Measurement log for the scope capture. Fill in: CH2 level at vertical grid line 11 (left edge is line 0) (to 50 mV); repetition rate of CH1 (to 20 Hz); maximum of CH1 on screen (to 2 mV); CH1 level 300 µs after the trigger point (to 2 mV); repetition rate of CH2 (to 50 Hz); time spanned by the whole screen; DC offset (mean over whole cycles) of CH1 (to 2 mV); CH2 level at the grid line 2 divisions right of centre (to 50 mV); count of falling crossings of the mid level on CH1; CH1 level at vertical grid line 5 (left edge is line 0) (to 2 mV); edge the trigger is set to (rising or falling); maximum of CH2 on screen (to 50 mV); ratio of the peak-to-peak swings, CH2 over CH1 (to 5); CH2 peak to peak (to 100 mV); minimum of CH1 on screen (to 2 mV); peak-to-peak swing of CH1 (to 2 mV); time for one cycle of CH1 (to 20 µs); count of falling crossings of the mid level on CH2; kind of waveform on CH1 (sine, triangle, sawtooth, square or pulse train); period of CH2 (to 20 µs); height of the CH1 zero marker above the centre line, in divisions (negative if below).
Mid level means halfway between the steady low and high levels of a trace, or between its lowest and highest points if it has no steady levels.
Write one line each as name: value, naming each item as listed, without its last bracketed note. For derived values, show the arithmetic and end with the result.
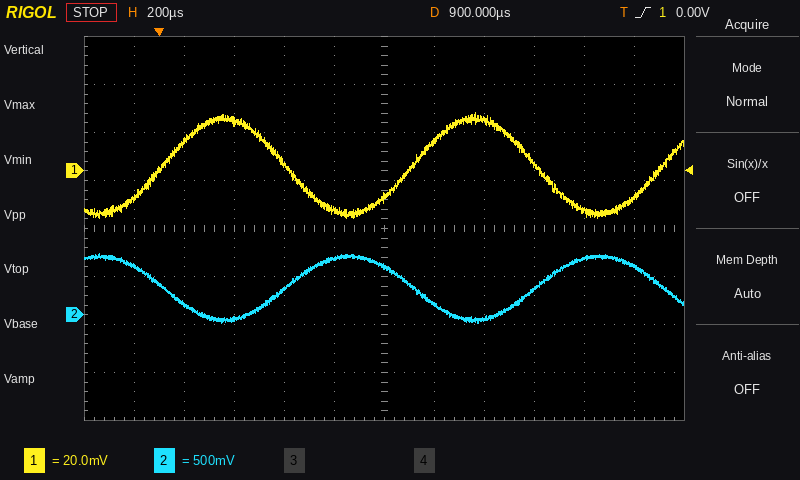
CH2 level at vertical grid line 11 (left edge is line 0): 500 mV
repetition rate of CH1: 1 / 1.00 ms ≈ 1.00 kHz
maximum of CH1 on screen: 24 mV
CH1 level 300 µs after the trigger point: 20 mV
repetition rate of CH2: 1 / 1.00 ms ≈ 1.00 kHz
time spanned by the whole screen: 2.4 ms
DC offset (mean over whole cycles) of CH1: (24 mV + (-20 mV)) / 2 ≈ 2 mV
CH2 level at the grid line 2 divisions right of centre: -50 mV
count of falling crossings of the mid level on CH1: 2
CH1 level at vertical grid line 5 (left edge is line 0): -16 mV
edge the trigger is set to: rising
maximum of CH2 on screen: 650 mV
ratio of the peak-to-peak swings, CH2 over CH1: 700 mV / 44 mV ≈ 15.9, so 15 to the nearest 5
CH2 peak to peak: 700 mV
minimum of CH1 on screen: -20 mV
peak-to-peak swing of CH1: 24 mV − (-20 mV) = 44 mV
time for one cycle of CH1: 1.00 ms
count of falling crossings of the mid level on CH2: 3
kind of waveform on CH1: sine
period of CH2: 1.00 ms
height of the CH1 zero marker above the centre line, in divisions: +1.2 div
